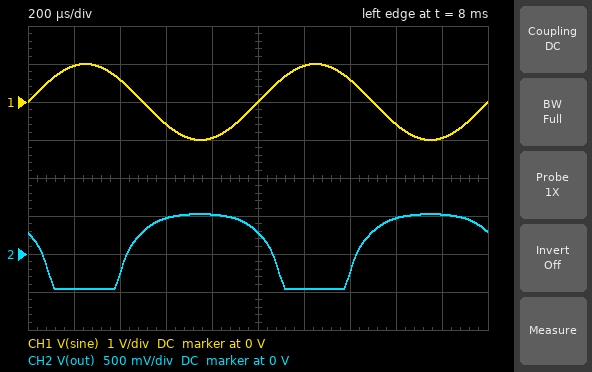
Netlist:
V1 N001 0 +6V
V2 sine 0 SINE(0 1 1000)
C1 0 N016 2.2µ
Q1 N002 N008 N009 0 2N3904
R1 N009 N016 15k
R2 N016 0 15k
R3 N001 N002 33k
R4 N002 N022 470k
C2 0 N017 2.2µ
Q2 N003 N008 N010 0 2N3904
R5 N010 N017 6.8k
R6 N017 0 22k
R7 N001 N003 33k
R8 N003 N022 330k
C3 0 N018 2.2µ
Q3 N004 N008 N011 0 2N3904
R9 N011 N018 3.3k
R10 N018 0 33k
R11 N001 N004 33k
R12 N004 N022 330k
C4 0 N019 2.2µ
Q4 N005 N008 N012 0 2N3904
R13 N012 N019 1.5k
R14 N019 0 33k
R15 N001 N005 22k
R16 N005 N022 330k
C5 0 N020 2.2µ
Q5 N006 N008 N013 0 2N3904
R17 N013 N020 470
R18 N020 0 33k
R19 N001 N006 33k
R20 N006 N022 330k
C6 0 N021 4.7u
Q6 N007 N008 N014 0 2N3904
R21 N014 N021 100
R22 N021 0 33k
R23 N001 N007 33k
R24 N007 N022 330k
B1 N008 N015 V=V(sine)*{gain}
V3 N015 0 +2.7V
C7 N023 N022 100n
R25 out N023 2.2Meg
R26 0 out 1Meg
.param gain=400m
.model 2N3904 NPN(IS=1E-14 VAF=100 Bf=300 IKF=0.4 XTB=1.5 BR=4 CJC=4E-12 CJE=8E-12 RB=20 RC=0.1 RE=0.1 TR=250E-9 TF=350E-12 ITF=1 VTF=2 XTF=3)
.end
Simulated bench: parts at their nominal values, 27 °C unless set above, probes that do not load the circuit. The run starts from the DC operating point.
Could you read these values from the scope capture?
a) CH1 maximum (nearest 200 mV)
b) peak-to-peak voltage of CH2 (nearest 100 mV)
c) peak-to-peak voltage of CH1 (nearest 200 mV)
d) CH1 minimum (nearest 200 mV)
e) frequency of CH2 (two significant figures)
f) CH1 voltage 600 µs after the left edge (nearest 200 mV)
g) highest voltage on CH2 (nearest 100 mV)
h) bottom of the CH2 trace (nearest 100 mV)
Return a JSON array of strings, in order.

["1.0 V", "1.0 V", "2.0 V", "-1.0 V", "1.0 kHz", "-600 mV", "500 mV", "-500 mV"]
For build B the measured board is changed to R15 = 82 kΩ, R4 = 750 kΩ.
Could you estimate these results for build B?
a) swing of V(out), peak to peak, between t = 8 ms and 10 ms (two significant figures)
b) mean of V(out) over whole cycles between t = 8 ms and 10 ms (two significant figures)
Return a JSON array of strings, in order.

["1.0 V", "230 mV"]
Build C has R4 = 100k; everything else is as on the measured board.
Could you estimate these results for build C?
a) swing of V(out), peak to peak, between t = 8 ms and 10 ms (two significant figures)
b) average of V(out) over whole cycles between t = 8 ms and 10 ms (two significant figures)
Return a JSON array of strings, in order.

["870 mV", "81 mV"]
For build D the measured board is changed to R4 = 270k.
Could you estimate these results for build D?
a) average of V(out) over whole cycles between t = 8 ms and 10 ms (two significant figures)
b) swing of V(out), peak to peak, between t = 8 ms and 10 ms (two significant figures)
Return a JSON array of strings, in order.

["100 mV", "950 mV"]
